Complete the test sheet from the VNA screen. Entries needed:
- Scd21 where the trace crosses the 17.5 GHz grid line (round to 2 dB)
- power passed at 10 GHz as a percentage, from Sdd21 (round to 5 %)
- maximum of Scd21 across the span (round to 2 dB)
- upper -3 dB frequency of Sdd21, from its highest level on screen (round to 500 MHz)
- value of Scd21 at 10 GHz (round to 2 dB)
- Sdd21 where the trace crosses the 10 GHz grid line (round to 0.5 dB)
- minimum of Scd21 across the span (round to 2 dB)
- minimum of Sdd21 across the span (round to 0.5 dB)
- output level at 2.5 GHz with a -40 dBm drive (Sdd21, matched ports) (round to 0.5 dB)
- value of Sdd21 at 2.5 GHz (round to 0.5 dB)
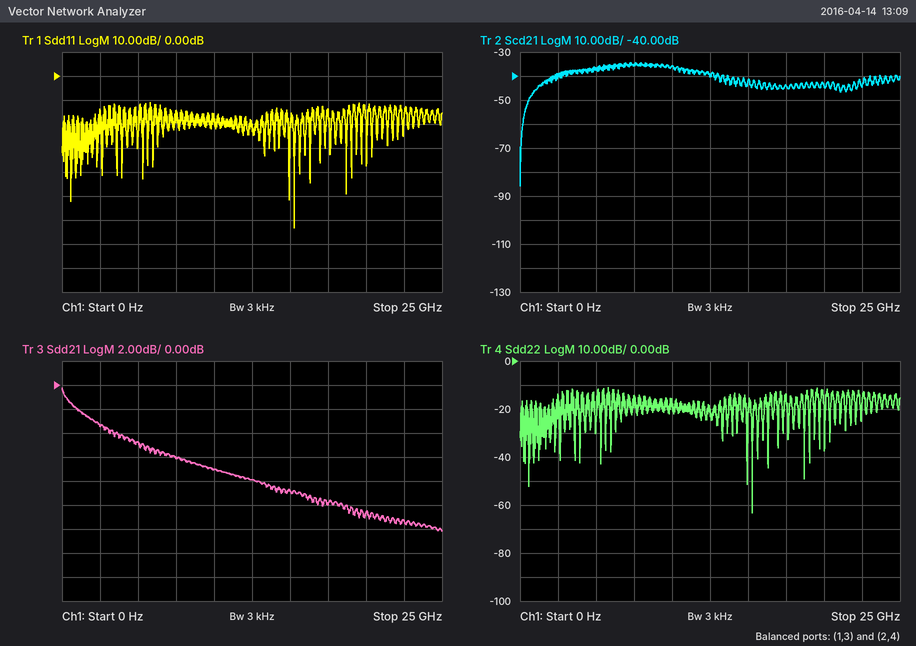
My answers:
-44 dB
20 %
-34 dB
2.5 GHz
-36 dB
-7.0 dB
-86 dB
-12.0 dB
-43.5 dBm
-3.5 dB
